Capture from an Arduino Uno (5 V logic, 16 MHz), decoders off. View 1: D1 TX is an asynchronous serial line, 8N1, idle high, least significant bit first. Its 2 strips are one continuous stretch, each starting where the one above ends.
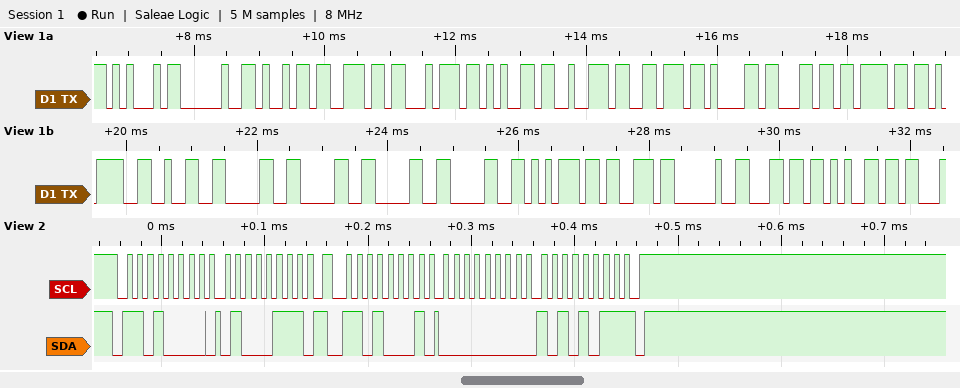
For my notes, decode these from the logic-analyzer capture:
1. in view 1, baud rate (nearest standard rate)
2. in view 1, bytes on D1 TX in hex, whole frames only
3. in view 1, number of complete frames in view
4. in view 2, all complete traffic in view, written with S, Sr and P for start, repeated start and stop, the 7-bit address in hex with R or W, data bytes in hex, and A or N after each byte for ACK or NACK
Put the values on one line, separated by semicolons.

9600 baud; 0x45 0x20 0x69 0x6E 0x74 0x65 0x72 0x76 0x61 0x6C 0x6F 0x3D 0x32 0x30 0x30 0x30 0x30 0x75 0x73 0x20 0x6C 0x65; 22; S 68W A 47 A Sr 68R A 00 A AB N P
